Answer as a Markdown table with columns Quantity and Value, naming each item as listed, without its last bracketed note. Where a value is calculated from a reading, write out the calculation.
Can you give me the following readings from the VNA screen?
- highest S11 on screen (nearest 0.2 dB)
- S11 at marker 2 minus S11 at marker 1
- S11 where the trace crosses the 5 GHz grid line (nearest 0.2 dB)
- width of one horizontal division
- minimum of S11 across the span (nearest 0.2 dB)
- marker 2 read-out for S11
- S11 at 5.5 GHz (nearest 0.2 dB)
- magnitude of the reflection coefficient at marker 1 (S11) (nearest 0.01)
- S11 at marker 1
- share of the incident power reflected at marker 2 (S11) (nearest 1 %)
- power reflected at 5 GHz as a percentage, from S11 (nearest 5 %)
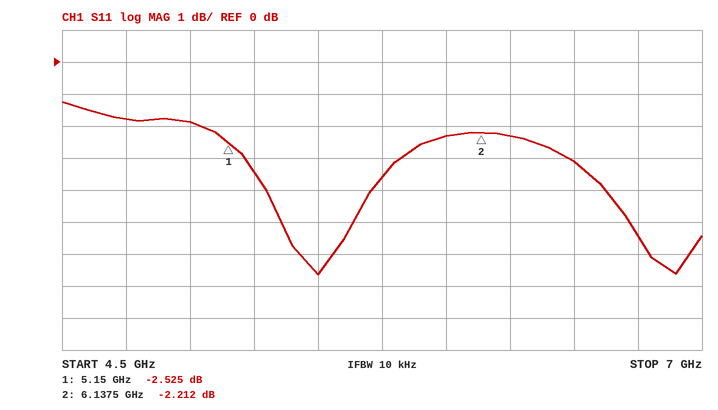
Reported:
| Quantity | Value |
|---|---|
| highest S11 on screen | -1.2 dB |
| S11 at marker 2 minus S11 at marker 1 | -2.212 − (-2.525) = 0.313 dB |
| S11 where the trace crosses the 5 GHz grid line | -1.8 dB |
| width of one horizontal division | 250 MHz |
| minimum of S11 across the span | -6.6 dB |
| marker 2 read-out for S11 | -2.212 dB |
| S11 at 5.5 GHz | -6.6 dB |
| magnitude of the reflection coefficient at marker 1 (S11) | 10^(-2.525/20) ≈ 0.75 |
| S11 at marker 1 | -2.525 dB |
| share of the incident power reflected at marker 2 (S11) | 10^(-2.212/10) ≈ 60 % |
| power reflected at 5 GHz as a percentage, from S11 | 10^(-1.8/10) ≈ 66.1 %, so 65 % to the nearest 5 % |
